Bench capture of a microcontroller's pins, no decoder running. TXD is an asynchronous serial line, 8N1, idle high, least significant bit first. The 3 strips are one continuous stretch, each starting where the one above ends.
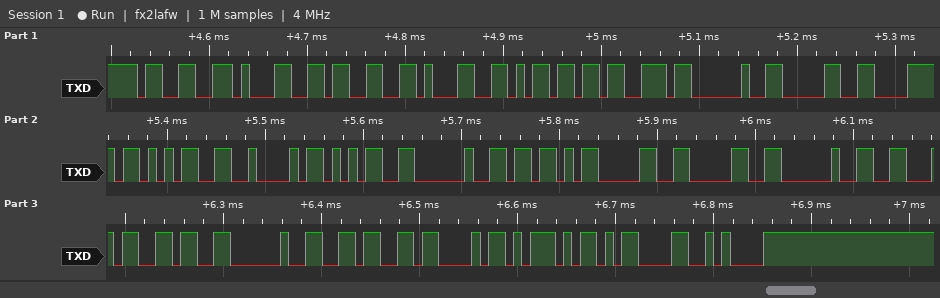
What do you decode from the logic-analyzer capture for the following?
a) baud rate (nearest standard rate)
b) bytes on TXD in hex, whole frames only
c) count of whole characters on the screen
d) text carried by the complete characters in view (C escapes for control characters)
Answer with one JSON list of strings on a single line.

["115200 baud", "33 31 33 31 6D 73 20 30 78 35 42 35 20 5B 30 30 20 46 36 20 36 43 5D 0D 0A", "25", "\"3131ms 0x5B5 [00 F6 6C]\\r\\n\""]
